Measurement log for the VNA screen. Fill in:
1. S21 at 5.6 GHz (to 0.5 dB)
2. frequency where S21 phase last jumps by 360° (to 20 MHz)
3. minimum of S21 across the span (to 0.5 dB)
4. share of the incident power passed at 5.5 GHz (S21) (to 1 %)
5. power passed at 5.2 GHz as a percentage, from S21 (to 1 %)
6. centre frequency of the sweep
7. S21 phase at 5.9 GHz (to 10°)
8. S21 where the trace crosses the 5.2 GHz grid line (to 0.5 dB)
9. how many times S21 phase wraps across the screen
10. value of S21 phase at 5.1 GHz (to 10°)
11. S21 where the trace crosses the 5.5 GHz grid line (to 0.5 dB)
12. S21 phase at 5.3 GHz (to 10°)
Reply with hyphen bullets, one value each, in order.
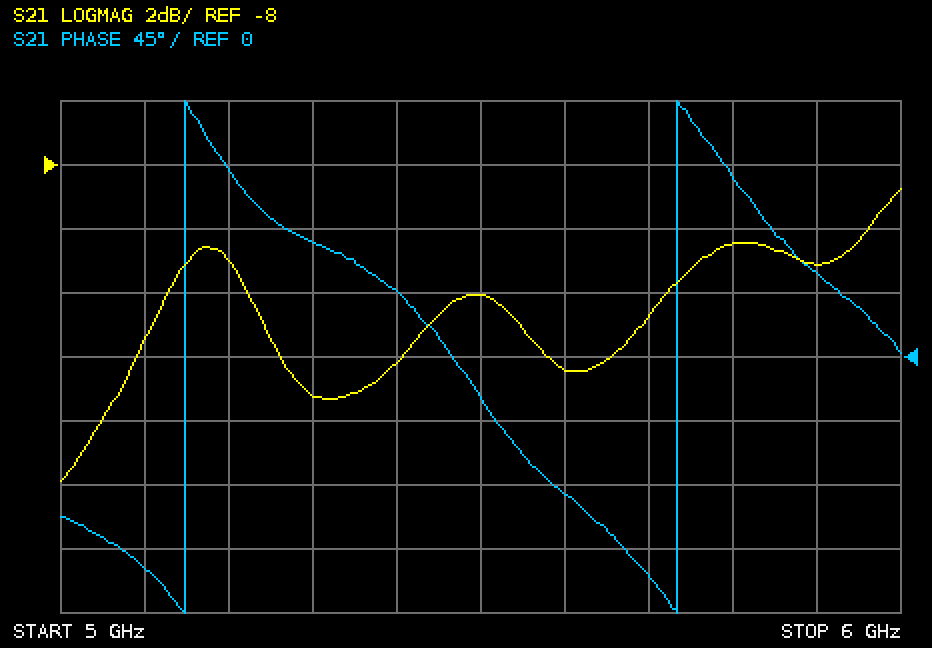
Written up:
- -14.5 dB
- 5.74 GHz
- -18.0 dB
- 6 %
- 8 %
- 5.5 GHz
- 60°
- -11.0 dB
- 2
- -150°
- -12.0 dB
- 80°
